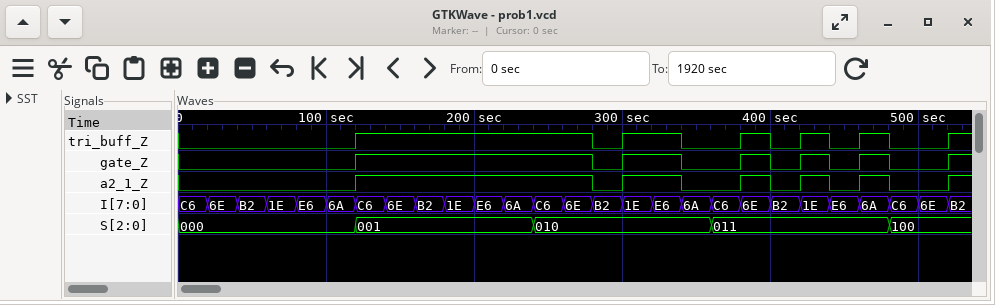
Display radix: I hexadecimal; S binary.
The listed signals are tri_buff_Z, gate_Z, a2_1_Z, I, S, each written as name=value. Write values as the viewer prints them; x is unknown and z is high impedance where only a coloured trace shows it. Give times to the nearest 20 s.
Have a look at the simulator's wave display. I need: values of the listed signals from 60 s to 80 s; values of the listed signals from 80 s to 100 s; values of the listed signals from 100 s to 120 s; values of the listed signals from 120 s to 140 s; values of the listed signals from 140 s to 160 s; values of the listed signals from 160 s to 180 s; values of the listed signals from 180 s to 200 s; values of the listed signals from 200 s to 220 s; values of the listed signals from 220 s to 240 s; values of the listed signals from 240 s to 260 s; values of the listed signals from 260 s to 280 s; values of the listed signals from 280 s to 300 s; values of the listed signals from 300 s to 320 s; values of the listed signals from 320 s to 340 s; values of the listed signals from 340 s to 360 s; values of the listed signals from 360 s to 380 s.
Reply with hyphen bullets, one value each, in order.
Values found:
- tri_buff_Z=0, gate_Z=0, a2_1_Z=0, I=1E, S=000
- tri_buff_Z=0, gate_Z=0, a2_1_Z=0, I=E6, S=000
- tri_buff_Z=0, gate_Z=0, a2_1_Z=0, I=6A, S=000
- tri_buff_Z=1, gate_Z=1, a2_1_Z=1, I=C6, S=001
- tri_buff_Z=1, gate_Z=1, a2_1_Z=1, I=6E, S=001
- tri_buff_Z=1, gate_Z=1, a2_1_Z=1, I=B2, S=001
- tri_buff_Z=1, gate_Z=1, a2_1_Z=1, I=1E, S=001
- tri_buff_Z=1, gate_Z=1, a2_1_Z=1, I=E6, S=001
- tri_buff_Z=1, gate_Z=1, a2_1_Z=1, I=6A, S=001
- tri_buff_Z=1, gate_Z=1, a2_1_Z=1, I=C6, S=010
- tri_buff_Z=1, gate_Z=1, a2_1_Z=1, I=6E, S=010
- tri_buff_Z=0, gate_Z=0, a2_1_Z=0, I=B2, S=010
- tri_buff_Z=1, gate_Z=1, a2_1_Z=1, I=1E, S=010
- tri_buff_Z=1, gate_Z=1, a2_1_Z=1, I=E6, S=010
- tri_buff_Z=0, gate_Z=0, a2_1_Z=0, I=6A, S=010
- tri_buff_Z=0, gate_Z=0, a2_1_Z=0, I=C6, S=011
